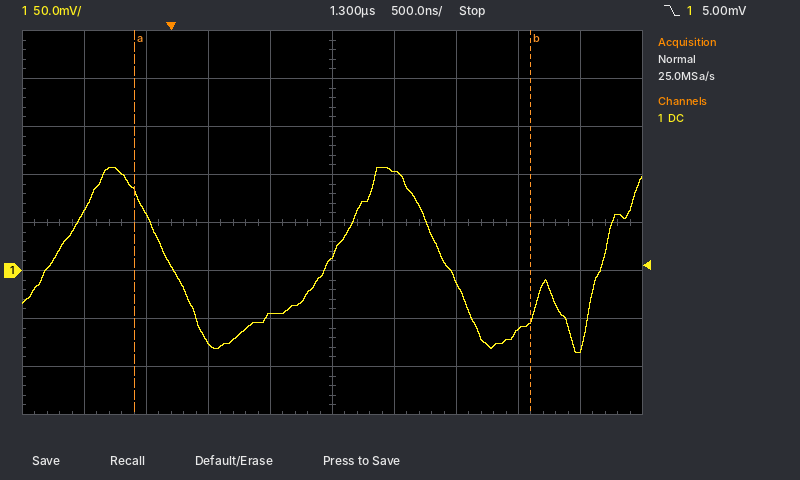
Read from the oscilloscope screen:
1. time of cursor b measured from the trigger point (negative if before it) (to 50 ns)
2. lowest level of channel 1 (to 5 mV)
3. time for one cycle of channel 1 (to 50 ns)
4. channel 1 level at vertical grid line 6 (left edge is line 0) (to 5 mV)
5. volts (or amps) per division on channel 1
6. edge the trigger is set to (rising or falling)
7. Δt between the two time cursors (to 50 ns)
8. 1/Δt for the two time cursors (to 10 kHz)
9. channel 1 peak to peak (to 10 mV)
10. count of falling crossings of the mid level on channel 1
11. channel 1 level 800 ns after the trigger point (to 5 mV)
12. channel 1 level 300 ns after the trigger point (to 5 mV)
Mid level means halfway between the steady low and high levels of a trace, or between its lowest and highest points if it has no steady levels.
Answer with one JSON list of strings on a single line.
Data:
["+2.90 µs", "-85 mV", "2.20 µs", "105 mV", "50 mV", "falling", "3.20 µs", "310 kHz", "190 mV", "2", "-45 mV", "-75 mV"]
